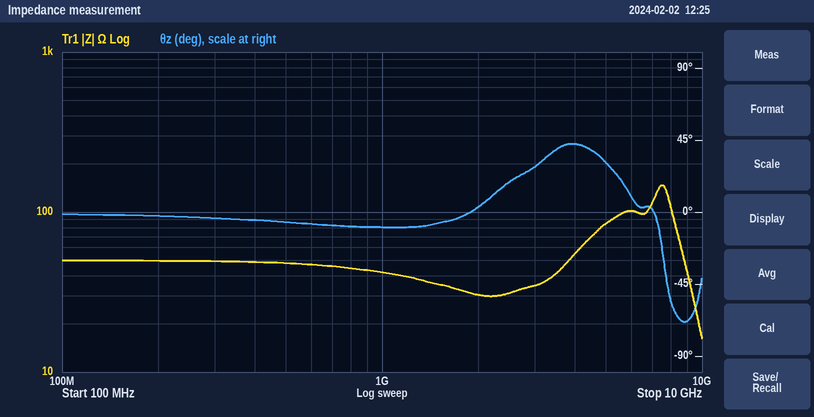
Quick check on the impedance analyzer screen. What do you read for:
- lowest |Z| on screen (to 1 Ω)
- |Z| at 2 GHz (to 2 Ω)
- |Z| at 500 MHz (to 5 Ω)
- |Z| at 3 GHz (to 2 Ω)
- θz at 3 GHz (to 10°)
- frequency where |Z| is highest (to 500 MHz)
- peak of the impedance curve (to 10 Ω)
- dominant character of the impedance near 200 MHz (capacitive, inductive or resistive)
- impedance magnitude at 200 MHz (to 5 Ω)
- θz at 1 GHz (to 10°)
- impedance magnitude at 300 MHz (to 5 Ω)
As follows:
16 Ω
30 Ω
50 Ω
34 Ω
30°
7.5 GHz
150 Ω
resistive
50 Ω
-10°
50 Ω
